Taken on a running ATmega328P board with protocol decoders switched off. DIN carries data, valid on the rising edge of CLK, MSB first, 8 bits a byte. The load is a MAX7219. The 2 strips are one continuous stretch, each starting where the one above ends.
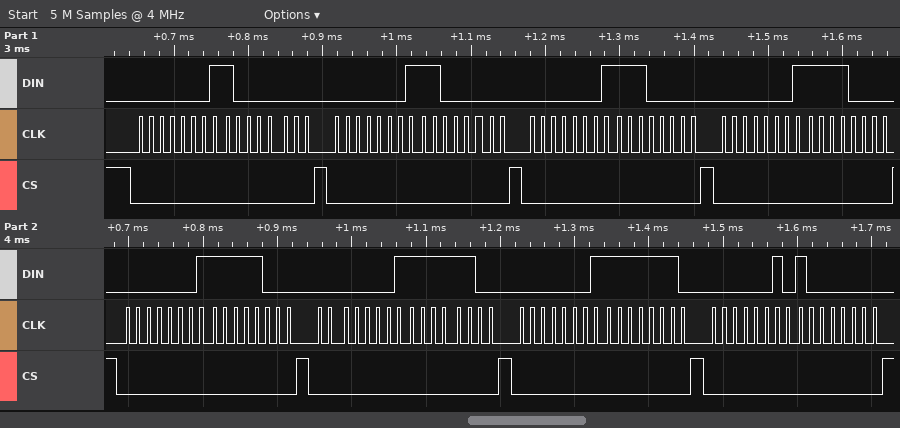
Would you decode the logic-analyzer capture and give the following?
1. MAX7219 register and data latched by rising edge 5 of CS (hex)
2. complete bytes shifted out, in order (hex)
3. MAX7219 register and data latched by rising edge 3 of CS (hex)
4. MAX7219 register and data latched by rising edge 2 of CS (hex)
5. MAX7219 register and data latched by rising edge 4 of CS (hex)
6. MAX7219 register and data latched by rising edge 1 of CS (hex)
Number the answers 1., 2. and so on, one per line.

1. register 0x1, data 0xF8
2. 01 80 01 C0 01 E0 01 F0 01 F8 01 FC 01 FE 02 80
3. register 0x1, data 0xE0
4. register 0x1, data 0xC0
5. register 0x1, data 0xF0
6. register 0x1, data 0x80
